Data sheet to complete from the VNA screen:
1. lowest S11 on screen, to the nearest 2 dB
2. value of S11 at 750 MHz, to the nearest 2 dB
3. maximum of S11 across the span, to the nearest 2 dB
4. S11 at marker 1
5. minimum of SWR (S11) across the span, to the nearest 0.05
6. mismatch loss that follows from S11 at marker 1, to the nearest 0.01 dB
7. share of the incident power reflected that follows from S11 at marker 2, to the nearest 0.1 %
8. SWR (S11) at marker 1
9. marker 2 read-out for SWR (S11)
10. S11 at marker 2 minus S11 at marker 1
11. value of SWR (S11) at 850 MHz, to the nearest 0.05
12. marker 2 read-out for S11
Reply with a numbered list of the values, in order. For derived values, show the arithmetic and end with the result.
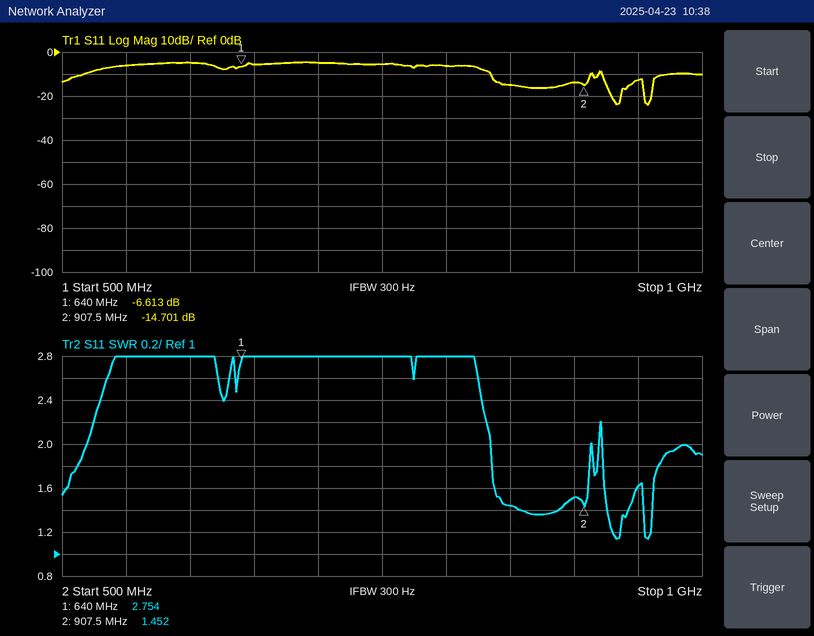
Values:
1. -24 dB
2. -6 dB
3. -4 dB
4. -6.613 dB
5. 1.15
6. −10 log10(1 − 10^(-6.613/10)) ≈ 1.07 dB
7. 10^(-14.701/10) ≈ 3.4 %
8. 2.754
9. 1.452
10. -14.701 − (-6.613) = -8.088 dB
11. 1.45
12. -14.701 dB
